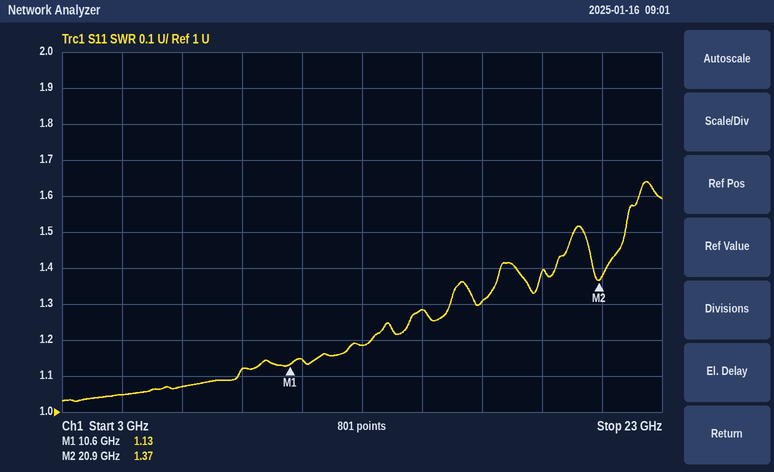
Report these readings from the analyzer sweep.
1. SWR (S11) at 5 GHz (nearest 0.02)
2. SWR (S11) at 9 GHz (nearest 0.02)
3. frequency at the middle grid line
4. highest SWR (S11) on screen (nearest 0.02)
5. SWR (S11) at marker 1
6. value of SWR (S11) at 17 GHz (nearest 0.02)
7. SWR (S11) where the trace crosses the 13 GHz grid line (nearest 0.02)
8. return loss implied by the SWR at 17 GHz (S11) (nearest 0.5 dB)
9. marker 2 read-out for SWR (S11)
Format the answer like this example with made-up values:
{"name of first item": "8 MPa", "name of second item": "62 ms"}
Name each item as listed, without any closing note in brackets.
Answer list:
{"SWR (S11) at 5 GHz": "1.04", "SWR (S11) at 9 GHz": "1.12", "frequency at the middle grid line": "13 GHz", "highest SWR (S11) on screen": "1.64", "SWR (S11) at marker 1": "1.13", "value of SWR (S11) at 17 GHz": "1.30", "SWR (S11) where the trace crosses the 13 GHz grid line": "1.18", "return loss implied by the SWR at 17 GHz (S11)": "17.5 dB", "marker 2 read-out for SWR": "1.37"}
